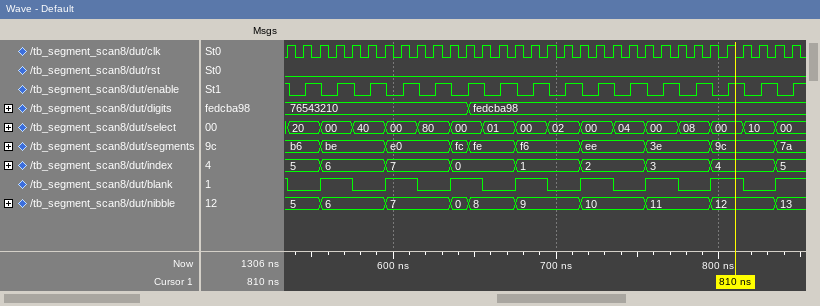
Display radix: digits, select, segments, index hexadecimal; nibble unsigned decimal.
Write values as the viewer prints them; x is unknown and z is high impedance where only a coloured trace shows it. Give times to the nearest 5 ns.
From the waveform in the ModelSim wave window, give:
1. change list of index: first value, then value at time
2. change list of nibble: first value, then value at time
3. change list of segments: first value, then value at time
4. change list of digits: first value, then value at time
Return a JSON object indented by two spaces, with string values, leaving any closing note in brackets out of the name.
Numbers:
{
  "change list of index: first value, then value at time": "5, 6 at 555 ns, 7 at 595 ns, 0 at 635 ns, 1 at 675 ns, 2 at 715 ns, 3 at 755 ns, 4 at 795 ns, 5 at 835 ns",
  "change list of nibble: first value, then value at time": "5, 6 at 555 ns, 7 at 595 ns, 0 at 635 ns, 8 at 645 ns, 9 at 675 ns, 10 at 715 ns, 11 at 755 ns, 12 at 795 ns, 13 at 835 ns",
  "change list of segments: first value, then value at time": "b6, be at 555 ns, e0 at 595 ns, fc at 635 ns, fe at 645 ns, f6 at 675 ns, ee at 715 ns, 3e at 755 ns, 9c at 795 ns, 7a at 835 ns",
  "change list of digits: first value, then value at time": "76543210, fedcba98 at 645 ns"
}
